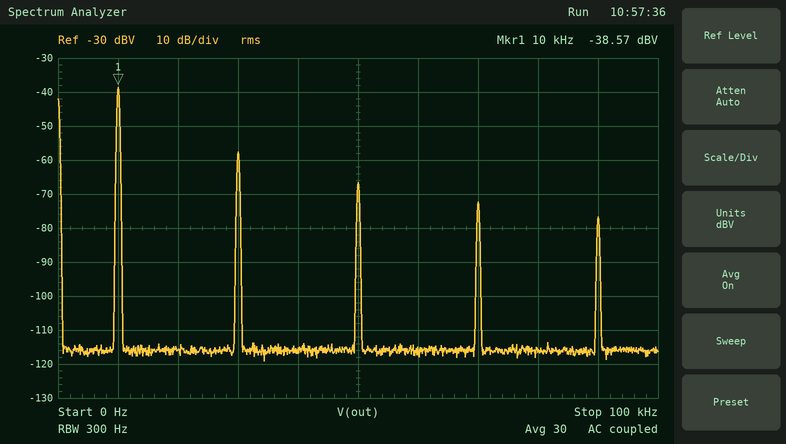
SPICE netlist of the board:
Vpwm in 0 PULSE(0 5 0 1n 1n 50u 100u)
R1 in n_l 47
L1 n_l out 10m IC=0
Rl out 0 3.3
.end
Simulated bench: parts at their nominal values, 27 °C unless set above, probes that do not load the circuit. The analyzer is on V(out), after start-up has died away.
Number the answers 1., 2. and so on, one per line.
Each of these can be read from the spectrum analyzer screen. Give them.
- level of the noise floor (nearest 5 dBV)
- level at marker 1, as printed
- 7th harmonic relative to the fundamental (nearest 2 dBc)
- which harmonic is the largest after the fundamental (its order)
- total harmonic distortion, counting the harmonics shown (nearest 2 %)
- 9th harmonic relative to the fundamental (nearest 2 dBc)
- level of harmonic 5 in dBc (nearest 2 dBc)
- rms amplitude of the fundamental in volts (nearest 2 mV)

1. -115 dBV
2. -38.57 dBV
3. -34 dBc
4. 3
5. 12 %
6. -38 dBc
7. -28 dBc
8. 12 mV
